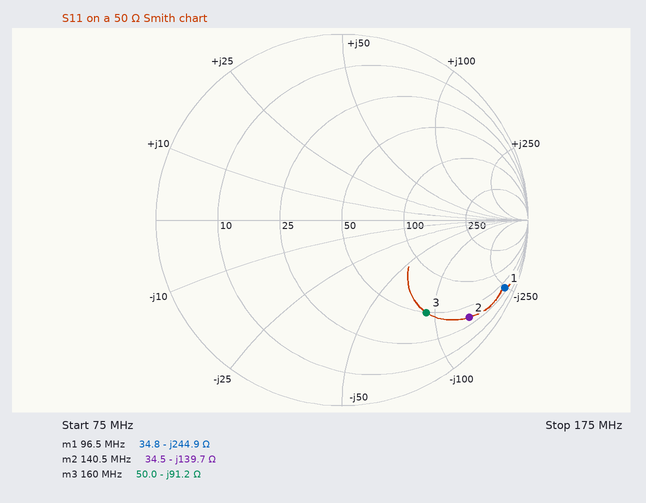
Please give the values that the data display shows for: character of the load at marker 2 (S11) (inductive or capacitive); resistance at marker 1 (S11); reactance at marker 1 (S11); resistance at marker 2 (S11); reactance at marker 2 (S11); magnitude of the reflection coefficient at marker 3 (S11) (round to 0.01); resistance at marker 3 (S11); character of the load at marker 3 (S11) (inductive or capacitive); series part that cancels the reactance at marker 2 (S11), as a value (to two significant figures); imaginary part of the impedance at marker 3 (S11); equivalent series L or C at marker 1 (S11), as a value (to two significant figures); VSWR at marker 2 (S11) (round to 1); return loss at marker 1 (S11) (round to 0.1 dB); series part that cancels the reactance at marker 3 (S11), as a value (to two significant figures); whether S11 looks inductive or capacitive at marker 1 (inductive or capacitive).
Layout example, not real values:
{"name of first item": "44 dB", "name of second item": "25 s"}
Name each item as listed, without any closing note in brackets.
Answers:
{"character of the load at marker 2 (S11)": "capacitive", "resistance at marker 1": "34.8 Ω", "reactance at marker 1": "-244.9 Ω", "resistance at marker 2": "34.5 Ω", "reactance at marker 2": "-139.7 Ω", "magnitude of the reflection coefficient at marker 3 (S11)": "0.67", "resistance at marker 3": "50.0 Ω", "character of the load at marker 3 (S11)": "capacitive", "series part that cancels the reactance at marker 2 (S11), as a value": "160 nH", "imaginary part of the impedance at marker 3": "-91.2 Ω", "equivalent series L or C at marker 1 (S11), as a value": "6.7 pF", "VSWR at marker 2 (S11)": "13", "return loss at marker 1 (S11)": "0.5 dB", "series part that cancels the reactance at marker 3 (S11), as a value": "91 nH", "whether S11 looks inductive or capacitive at marker 1": "capacitive"}
